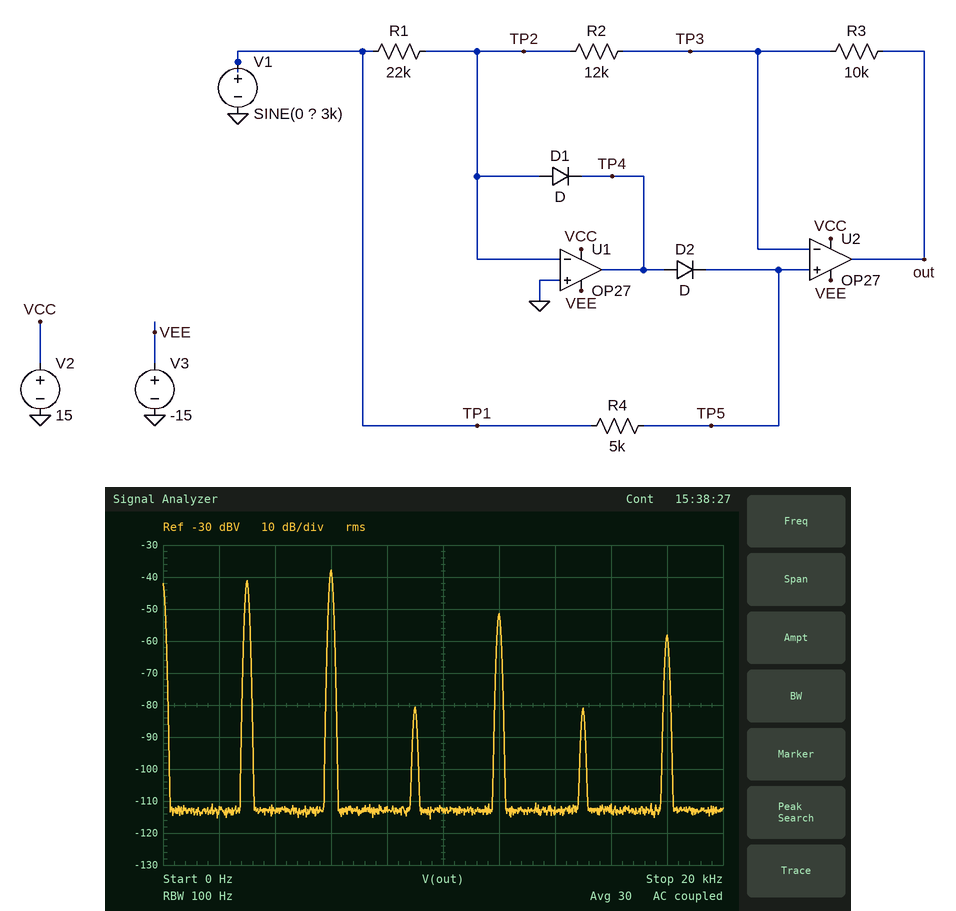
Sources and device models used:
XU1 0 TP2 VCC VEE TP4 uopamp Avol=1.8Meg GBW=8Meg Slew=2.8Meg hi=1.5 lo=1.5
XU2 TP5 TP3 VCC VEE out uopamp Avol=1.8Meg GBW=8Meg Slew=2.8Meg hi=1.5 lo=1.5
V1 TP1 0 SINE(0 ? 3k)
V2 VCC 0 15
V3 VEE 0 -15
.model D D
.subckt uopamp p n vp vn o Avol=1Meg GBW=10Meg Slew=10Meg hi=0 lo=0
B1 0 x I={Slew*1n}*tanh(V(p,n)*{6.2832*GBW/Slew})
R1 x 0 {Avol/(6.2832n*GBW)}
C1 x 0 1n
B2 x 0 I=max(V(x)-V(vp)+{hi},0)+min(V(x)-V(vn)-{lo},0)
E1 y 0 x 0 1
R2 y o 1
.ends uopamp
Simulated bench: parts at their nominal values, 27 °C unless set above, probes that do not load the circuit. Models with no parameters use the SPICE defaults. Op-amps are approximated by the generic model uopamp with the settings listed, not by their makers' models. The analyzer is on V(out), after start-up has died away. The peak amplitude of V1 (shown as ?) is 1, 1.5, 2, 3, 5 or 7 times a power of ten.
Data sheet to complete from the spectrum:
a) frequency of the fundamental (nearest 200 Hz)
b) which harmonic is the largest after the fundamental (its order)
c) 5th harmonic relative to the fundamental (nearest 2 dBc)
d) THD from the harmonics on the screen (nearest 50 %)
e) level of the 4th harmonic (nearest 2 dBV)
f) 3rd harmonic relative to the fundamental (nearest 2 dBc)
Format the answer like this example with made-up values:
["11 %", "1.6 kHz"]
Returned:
["3.0 kHz", "2", "-40 dBc", "150 %", "-52 dBV", "-40 dBc"]
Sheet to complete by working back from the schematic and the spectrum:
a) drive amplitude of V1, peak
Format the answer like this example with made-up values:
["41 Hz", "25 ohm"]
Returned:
["30 mV"]
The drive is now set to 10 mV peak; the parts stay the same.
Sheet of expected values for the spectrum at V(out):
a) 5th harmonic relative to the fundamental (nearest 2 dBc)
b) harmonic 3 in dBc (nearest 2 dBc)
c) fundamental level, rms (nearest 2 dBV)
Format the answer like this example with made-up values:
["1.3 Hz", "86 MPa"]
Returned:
["-32 dBc", "-30 dBc", "-50 dBV"]
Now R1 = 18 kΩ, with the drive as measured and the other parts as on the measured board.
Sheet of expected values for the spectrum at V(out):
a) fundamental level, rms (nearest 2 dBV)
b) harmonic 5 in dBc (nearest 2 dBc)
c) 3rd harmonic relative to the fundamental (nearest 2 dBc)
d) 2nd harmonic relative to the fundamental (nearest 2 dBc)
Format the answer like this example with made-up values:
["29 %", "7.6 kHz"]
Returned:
["-44 dBV", "-36 dBc", "-36 dBc", "6 dBc"]
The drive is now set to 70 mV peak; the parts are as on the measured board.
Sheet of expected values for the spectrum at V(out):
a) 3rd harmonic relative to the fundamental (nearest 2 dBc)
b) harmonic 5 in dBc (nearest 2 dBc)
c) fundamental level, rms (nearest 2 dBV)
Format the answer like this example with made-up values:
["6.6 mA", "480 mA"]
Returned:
["-46 dBc", "-46 dBc", "-34 dBV"]
